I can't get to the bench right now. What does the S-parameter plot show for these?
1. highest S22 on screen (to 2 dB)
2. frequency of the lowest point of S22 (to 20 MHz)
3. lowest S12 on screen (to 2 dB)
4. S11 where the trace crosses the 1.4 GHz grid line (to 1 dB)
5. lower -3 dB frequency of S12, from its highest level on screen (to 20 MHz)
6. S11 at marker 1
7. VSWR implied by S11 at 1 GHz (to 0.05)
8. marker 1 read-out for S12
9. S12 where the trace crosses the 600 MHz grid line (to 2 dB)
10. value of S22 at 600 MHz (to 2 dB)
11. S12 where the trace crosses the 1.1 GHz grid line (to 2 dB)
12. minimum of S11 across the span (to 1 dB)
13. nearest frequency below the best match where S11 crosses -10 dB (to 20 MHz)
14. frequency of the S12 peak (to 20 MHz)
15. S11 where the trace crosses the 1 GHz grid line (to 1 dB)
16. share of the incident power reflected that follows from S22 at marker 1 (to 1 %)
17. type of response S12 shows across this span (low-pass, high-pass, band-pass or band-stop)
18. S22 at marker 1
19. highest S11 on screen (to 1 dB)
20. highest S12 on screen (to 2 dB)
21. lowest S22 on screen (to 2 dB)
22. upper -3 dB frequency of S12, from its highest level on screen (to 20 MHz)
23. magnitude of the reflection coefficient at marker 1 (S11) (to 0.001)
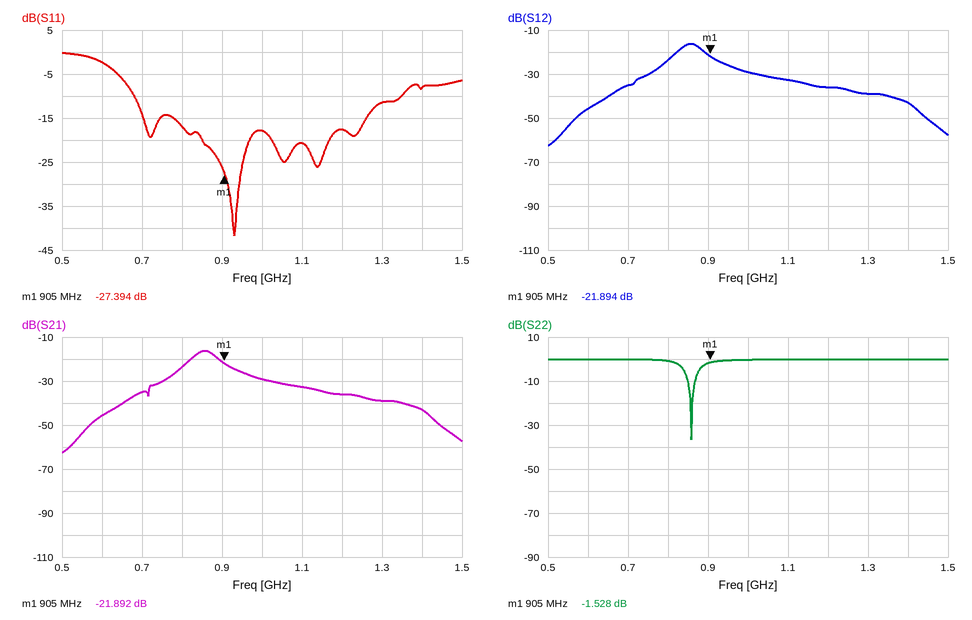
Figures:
0 dB
860 MHz
-62 dB
-8 dB
820 MHz
-27.394 dB
1.30
-21.894 dB
-46 dB
0 dB
-32 dB
-42 dB
680 MHz
860 MHz
-18 dB
70 %
band-pass
-1.528 dB
0 dB
-16 dB
-36 dB
880 MHz
0.043
